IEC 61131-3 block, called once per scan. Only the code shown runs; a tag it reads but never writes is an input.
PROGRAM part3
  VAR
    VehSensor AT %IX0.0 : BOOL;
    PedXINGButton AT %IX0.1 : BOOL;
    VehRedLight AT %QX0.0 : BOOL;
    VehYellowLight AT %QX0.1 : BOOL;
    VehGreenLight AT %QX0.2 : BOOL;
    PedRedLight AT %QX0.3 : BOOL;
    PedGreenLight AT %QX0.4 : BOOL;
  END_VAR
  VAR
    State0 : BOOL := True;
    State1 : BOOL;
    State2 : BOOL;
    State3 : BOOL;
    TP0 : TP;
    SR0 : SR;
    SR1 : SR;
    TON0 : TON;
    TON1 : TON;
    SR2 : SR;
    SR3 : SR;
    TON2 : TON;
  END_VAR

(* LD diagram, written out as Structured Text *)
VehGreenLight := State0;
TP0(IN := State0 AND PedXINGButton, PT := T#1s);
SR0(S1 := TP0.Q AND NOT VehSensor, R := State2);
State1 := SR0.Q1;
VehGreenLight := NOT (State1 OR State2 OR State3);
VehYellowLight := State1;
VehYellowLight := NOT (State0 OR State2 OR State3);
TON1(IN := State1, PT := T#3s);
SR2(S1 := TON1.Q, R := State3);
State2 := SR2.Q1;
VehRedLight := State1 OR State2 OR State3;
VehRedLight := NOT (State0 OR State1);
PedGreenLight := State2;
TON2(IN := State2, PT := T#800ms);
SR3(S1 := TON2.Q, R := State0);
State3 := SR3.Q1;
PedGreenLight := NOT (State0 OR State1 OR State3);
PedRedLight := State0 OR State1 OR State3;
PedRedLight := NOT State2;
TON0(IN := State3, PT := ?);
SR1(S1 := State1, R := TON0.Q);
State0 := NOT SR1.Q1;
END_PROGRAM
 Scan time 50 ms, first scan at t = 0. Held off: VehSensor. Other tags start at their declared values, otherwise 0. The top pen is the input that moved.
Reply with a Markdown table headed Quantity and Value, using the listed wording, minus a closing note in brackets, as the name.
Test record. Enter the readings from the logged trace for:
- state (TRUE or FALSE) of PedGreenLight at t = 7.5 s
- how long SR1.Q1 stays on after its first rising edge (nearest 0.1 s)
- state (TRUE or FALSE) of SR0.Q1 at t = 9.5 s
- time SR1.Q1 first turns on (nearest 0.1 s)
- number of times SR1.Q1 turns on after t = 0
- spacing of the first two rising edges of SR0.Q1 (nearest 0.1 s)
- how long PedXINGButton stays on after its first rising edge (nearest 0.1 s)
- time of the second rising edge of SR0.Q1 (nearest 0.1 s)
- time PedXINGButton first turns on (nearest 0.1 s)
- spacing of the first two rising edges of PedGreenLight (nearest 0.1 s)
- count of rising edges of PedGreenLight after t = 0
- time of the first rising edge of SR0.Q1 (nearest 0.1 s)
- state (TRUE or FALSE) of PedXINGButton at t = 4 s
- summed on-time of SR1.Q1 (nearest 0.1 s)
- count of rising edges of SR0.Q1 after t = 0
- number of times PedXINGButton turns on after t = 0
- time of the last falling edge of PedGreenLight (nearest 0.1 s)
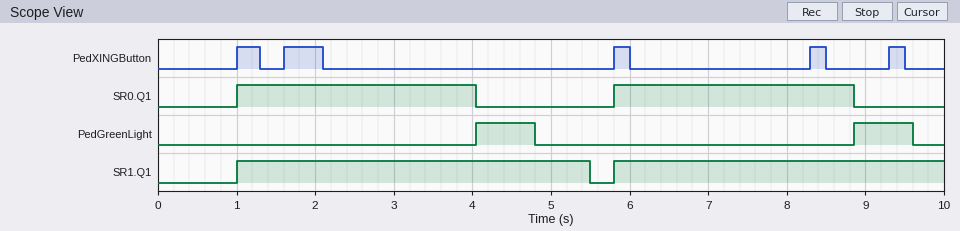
| Quantity | Value |
|---|---|
| state (TRUE or FALSE) of PedGreenLight at t = 7.5 s | FALSE |
| how long SR1.Q1 stays on after its first rising edge | 4.5 s |
| state (TRUE or FALSE) of SR0.Q1 at t = 9.5 s | FALSE |
| time SR1.Q1 first turns on | 1.0 s |
| number of times SR1.Q1 turns on after t = 0 | 2 |
| spacing of the first two rising edges of SR0.Q1 | 4.8 s |
| how long PedXINGButton stays on after its first rising edge | 0.3 s |
| time of the second rising edge of SR0.Q1 | 5.8 s |
| time PedXINGButton first turns on | 1.0 s |
| spacing of the first two rising edges of PedGreenLight | 4.8 s |
| count of rising edges of PedGreenLight after t = 0 | 2 |
| time of the first rising edge of SR0.Q1 | 1.0 s |
| state (TRUE or FALSE) of PedXINGButton at t = 4 s | FALSE |
| summed on-time of SR1.Q1 | 8.7 s |
| count of rising edges of SR0.Q1 after t = 0 | 2 |
| number of times PedXINGButton turns on after t = 0 | 5 |
| time of the last falling edge of PedGreenLight | 9.6 s |
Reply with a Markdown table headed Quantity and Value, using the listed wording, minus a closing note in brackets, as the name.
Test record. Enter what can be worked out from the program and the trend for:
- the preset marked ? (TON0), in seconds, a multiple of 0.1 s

| Quantity | Value |
|---|---|
| the preset marked ? (TON0), in seconds, a multiple of 0.1 s | 0.7 s |
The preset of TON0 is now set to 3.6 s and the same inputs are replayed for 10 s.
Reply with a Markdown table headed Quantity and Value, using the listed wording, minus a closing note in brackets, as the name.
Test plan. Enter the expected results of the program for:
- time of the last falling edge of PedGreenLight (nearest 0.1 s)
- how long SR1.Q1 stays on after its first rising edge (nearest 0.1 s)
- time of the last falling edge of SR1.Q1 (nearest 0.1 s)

| Quantity | Value |
|---|---|
| time of the last falling edge of PedGreenLight | 4.8 s |
| how long SR1.Q1 stays on after its first rising edge | 7.4 s |
| time of the last falling edge of SR1.Q1 | 8.4 s |
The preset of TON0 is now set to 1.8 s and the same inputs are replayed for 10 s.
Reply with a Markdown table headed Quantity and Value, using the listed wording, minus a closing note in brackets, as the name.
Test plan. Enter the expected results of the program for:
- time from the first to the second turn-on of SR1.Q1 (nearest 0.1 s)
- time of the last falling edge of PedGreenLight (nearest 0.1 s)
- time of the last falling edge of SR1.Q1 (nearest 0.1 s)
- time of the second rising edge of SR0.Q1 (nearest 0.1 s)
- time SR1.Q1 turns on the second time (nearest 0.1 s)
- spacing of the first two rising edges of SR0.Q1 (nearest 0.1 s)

| Quantity | Value |
|---|---|
| time from the first to the second turn-on of SR1.Q1 | 7.3 s |
| time of the last falling edge of PedGreenLight | 4.8 s |
| time of the last falling edge of SR1.Q1 | 6.6 s |
| time of the second rising edge of SR0.Q1 | 8.3 s |
| time SR1.Q1 turns on the second time | 8.3 s |
| spacing of the first two rising edges of SR0.Q1 | 7.3 s |
